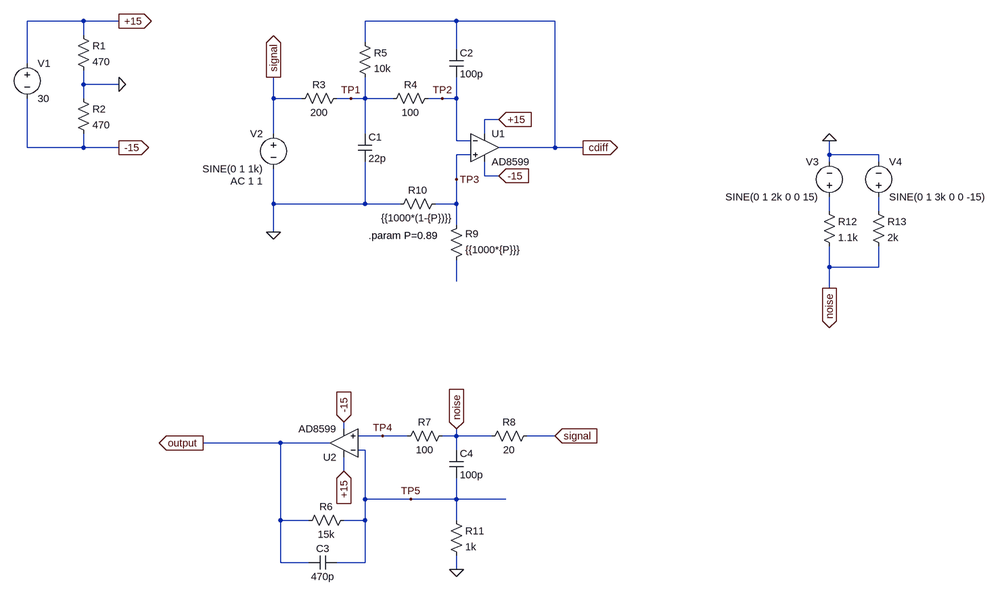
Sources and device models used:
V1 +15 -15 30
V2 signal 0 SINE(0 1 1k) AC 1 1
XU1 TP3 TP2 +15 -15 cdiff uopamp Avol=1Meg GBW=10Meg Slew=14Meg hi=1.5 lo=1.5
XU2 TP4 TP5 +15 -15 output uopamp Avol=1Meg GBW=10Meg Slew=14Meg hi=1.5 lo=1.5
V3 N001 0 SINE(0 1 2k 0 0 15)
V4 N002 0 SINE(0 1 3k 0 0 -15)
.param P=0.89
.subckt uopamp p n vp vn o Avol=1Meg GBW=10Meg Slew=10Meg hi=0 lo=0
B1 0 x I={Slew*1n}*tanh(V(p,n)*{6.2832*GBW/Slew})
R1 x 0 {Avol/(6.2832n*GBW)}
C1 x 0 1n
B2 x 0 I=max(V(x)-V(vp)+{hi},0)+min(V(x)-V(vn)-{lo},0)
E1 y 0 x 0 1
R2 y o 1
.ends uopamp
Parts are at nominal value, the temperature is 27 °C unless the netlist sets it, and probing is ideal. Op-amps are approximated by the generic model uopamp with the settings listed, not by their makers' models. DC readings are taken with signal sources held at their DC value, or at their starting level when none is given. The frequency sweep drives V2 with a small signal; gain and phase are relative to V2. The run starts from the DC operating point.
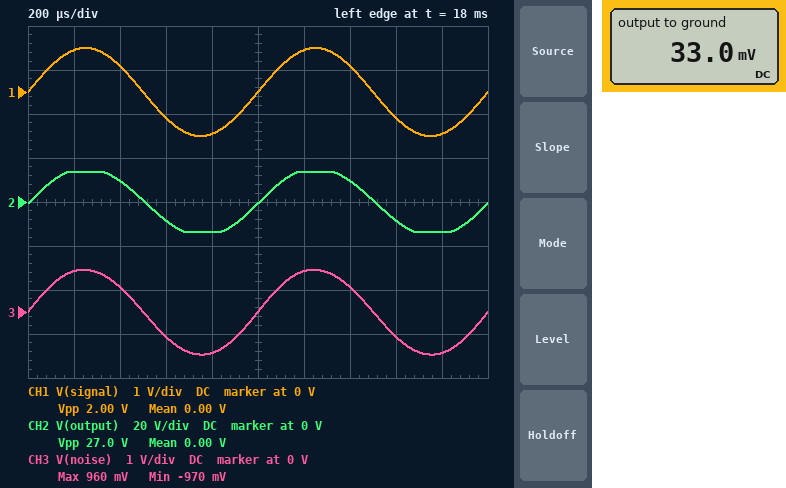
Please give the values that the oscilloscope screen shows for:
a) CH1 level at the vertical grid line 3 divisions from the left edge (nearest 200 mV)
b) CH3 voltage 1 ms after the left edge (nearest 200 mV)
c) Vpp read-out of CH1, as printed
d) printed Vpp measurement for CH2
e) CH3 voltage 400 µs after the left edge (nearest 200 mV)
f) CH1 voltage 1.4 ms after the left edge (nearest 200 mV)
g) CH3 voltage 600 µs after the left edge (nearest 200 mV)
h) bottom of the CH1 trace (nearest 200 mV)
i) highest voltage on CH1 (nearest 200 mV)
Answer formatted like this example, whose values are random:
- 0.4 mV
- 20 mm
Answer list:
- -600 mV
- 0 V
- 2.00 V
- 27.0 V
- 600 mV
- 600 mV
- -600 mV
- -1.0 V
- 1.0 V
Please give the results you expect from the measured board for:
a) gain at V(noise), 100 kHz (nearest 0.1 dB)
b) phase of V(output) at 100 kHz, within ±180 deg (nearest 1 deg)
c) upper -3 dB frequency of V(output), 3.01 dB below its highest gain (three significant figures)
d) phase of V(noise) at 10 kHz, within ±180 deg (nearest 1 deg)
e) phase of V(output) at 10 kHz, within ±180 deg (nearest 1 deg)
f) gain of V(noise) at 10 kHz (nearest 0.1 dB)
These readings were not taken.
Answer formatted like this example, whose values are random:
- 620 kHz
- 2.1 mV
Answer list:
- -0.2 dB
- -63 deg
- 21.9 kHz
- 0 deg
- -23 deg
- -0.2 dB
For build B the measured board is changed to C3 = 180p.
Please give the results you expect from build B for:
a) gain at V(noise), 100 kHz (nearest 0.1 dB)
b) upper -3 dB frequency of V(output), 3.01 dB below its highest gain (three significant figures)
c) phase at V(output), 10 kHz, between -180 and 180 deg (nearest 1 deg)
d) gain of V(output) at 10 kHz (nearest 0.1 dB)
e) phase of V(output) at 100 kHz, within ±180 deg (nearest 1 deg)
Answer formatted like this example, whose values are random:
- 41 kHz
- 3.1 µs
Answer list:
- -0.2 dB
- 54.5 kHz
- -10 deg
- 23.7 dB
- -56 deg
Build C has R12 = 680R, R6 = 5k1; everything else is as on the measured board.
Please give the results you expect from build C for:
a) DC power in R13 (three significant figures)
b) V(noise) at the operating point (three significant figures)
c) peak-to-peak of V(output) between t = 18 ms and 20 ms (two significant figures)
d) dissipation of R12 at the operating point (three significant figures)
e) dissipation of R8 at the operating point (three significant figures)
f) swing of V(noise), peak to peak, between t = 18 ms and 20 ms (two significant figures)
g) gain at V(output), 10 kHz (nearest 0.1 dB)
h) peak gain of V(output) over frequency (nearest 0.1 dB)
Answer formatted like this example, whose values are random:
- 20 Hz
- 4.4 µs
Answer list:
- 34.8 µW
- 4.83 mV
- 12 V
- 94.9 µW
- 1.17 µW
- 1.9 V
- 15.3 dB
- 15.4 dB
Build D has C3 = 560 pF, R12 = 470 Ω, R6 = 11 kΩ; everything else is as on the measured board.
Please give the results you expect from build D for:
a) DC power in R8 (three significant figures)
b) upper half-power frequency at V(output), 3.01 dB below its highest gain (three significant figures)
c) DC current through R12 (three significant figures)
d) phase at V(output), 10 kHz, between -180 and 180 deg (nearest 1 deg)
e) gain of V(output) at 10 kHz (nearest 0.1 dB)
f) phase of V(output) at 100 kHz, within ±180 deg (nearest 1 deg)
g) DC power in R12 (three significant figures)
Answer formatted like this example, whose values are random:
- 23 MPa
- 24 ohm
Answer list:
- 3.20 µW
- 25.3 kHz
- 534 µA
- -20 deg
- 20.5 dB
- -59 deg
- 134 µW
